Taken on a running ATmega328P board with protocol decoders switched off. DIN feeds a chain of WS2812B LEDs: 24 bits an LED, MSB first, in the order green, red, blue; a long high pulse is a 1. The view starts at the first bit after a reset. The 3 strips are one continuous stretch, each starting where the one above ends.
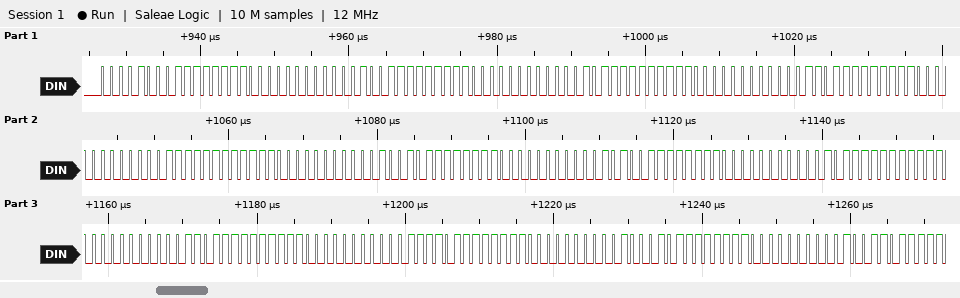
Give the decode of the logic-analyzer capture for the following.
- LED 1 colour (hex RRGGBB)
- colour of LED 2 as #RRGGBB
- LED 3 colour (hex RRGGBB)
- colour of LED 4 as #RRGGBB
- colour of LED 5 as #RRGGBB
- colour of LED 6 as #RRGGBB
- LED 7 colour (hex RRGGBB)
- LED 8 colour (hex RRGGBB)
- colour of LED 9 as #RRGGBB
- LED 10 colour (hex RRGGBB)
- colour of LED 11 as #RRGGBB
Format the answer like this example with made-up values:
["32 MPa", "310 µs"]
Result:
["#FF0800", "#FF0900", "#FF0B00", "#FF0D00", "#FF0F00", "#FF1200", "#FF1400", "#FF1700", "#FF1B00", "#FF1E00", "#FF2200"]
